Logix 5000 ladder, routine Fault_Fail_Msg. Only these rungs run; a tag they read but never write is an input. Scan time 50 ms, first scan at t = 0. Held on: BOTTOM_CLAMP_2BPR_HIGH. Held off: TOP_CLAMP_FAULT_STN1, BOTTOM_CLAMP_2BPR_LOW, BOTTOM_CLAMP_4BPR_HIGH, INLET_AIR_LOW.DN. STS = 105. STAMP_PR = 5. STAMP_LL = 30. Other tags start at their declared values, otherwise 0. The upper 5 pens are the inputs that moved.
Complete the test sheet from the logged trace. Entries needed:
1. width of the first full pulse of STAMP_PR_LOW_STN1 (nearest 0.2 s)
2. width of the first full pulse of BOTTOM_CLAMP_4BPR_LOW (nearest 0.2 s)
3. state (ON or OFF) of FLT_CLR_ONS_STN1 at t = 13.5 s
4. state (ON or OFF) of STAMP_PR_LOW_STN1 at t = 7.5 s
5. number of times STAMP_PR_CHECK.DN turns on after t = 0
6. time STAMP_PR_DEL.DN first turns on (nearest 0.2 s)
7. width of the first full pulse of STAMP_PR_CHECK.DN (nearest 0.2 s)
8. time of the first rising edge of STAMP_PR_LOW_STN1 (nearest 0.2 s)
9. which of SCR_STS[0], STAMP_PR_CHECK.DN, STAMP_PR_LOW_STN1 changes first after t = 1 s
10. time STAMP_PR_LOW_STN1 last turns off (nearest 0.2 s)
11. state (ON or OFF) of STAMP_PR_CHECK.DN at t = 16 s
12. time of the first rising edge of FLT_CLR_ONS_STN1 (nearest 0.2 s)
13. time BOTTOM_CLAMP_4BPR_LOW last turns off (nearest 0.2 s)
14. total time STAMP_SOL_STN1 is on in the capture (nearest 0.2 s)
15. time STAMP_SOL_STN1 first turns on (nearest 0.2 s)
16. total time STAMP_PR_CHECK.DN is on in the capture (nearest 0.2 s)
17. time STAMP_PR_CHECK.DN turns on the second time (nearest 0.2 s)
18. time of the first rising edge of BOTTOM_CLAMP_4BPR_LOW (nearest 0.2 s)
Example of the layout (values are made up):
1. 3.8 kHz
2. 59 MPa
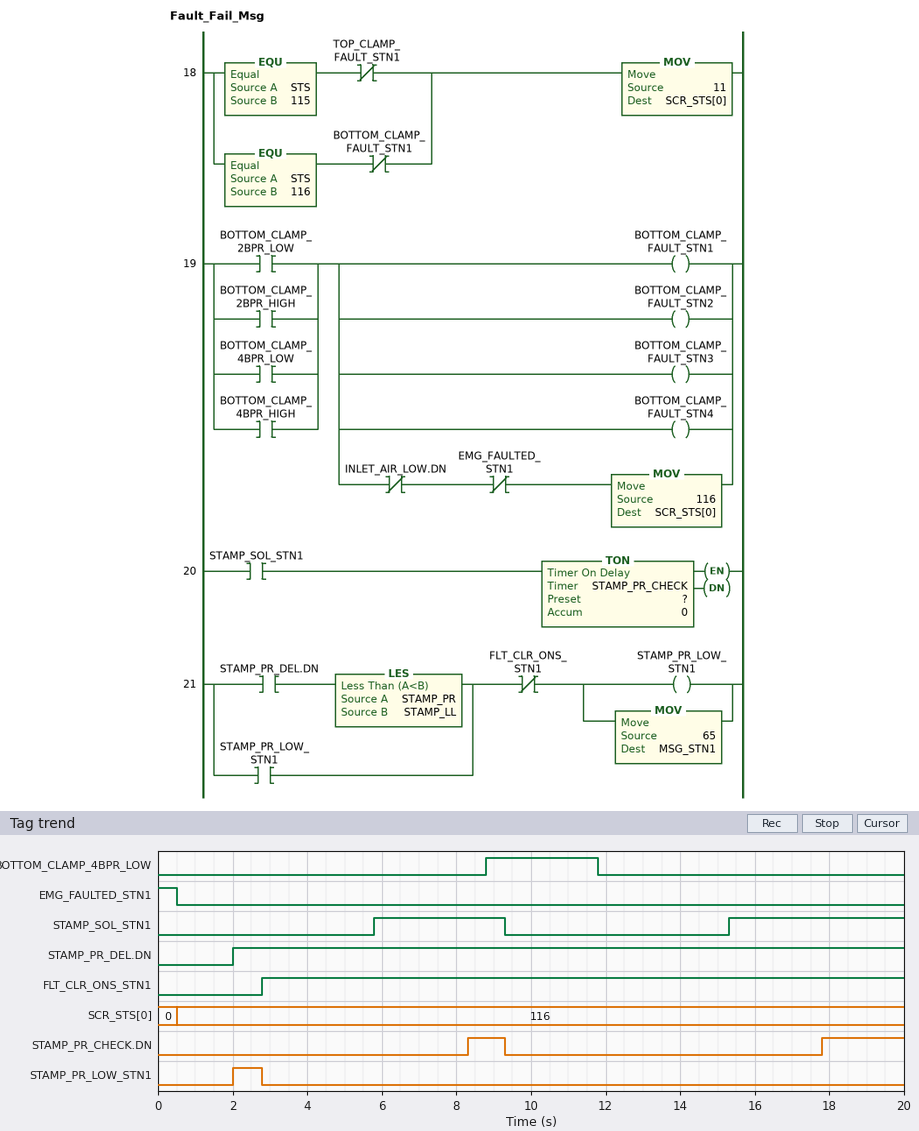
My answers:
1. 0.8 s
2. 3.0 s
3. ON
4. OFF
5. 2
6. 2.0 s
7. 1.0 s
8. 2.0 s
9. STAMP_PR_LOW_STN1
10. 2.8 s
11. OFF
12. 2.8 s
13. 11.8 s
14. 8.2 s
15. 5.8 s
16. 3.2 s
17. 17.8 s
18. 8.8 s
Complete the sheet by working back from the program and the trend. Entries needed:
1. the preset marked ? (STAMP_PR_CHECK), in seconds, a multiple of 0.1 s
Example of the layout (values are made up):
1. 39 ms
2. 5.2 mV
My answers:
1. 2.5 s
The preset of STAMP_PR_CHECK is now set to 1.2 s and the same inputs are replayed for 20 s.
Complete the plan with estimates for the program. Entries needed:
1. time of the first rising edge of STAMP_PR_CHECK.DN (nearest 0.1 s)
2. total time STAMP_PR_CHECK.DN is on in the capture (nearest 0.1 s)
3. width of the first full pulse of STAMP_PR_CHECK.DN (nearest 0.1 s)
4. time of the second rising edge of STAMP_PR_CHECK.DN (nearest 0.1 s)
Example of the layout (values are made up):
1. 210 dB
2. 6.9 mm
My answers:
1. 7.0 s
2. 5.8 s
3. 2.3 s
4. 16.5 s
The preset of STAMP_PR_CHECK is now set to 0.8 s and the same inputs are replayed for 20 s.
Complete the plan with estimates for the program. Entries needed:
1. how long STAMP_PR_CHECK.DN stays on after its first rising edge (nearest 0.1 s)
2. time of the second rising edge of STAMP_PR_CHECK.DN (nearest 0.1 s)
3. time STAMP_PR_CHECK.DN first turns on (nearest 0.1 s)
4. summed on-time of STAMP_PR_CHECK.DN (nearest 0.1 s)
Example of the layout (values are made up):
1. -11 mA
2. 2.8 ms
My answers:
1. 2.7 s
2. 16.1 s
3. 6.6 s
4. 6.6 s
